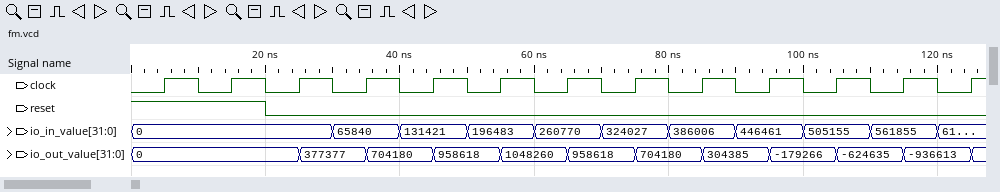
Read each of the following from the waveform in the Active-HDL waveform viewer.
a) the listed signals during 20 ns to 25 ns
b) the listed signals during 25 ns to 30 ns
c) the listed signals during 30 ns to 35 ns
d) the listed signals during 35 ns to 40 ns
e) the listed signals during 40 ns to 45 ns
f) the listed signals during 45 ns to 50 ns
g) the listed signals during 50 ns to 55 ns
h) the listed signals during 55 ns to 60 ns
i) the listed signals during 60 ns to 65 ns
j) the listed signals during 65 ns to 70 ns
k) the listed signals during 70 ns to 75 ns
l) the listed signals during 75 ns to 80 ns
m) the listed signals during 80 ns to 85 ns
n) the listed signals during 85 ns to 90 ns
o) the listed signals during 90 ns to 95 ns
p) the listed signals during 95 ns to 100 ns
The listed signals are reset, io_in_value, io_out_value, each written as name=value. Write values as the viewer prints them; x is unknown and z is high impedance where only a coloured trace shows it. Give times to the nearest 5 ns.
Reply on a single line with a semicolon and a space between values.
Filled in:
reset=0, io_in_value=0, io_out_value=0; reset=0, io_in_value=0, io_out_value=377377; reset=0, io_in_value=65840, io_out_value=377377; reset=0, io_in_value=65840, io_out_value=704180; reset=0, io_in_value=131421, io_out_value=704180; reset=0, io_in_value=131421, io_out_value=958618; reset=0, io_in_value=196483, io_out_value=958618; reset=0, io_in_value=196483, io_out_value=1048260; reset=0, io_in_value=260770, io_out_value=1048260; reset=0, io_in_value=260770, io_out_value=958618; reset=0, io_in_value=324027, io_out_value=958618; reset=0, io_in_value=324027, io_out_value=704180; reset=0, io_in_value=386006, io_out_value=704180; reset=0, io_in_value=386006, io_out_value=304385; reset=0, io_in_value=446461, io_out_value=304385; reset=0, io_in_value=446461, io_out_value=-179266
